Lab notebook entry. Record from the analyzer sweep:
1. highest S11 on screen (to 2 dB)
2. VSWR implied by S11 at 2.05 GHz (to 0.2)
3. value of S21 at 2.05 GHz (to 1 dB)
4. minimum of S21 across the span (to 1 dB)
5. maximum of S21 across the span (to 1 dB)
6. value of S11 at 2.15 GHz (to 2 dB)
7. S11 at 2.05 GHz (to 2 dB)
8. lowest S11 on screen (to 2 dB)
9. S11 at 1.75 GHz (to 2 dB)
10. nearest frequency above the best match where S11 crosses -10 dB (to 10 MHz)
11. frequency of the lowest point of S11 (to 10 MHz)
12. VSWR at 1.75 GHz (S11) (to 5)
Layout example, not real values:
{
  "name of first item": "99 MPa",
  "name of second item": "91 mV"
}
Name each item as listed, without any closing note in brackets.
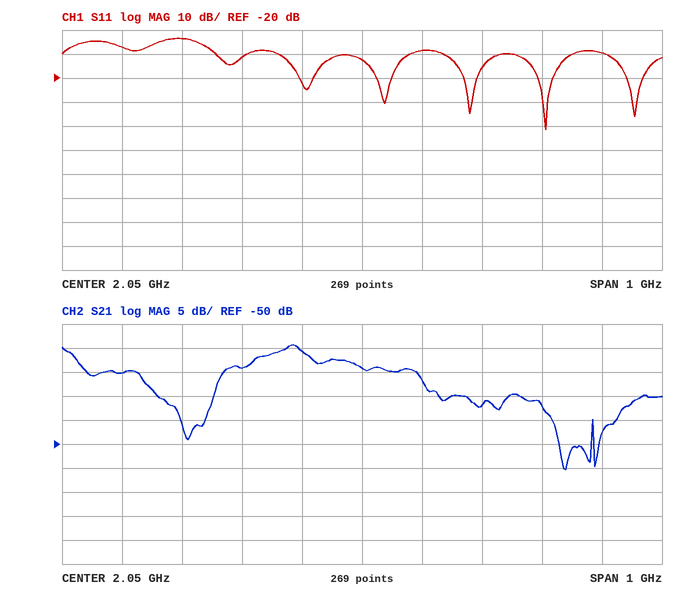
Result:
{
  "highest S11 on screen": "-4 dB",
  "VSWR implied by S11 at 2.05 GHz": "1.6",
  "value of S21 at 2.05 GHz": "-34 dB",
  "minimum of S21 across the span": "-55 dB",
  "maximum of S21 across the span": "-29 dB",
  "value of S11 at 2.15 GHz": "-8 dB",
  "S11 at 2.05 GHz": "-12 dB",
  "lowest S11 on screen": "-42 dB",
  "S11 at 1.75 GHz": "-4 dB",
  "nearest frequency above the best match where S11 crosses -10 dB": "2.40 GHz",
  "frequency of the lowest point of S11": "2.36 GHz",
  "VSWR at 1.75 GHz (S11)": "5"
}
